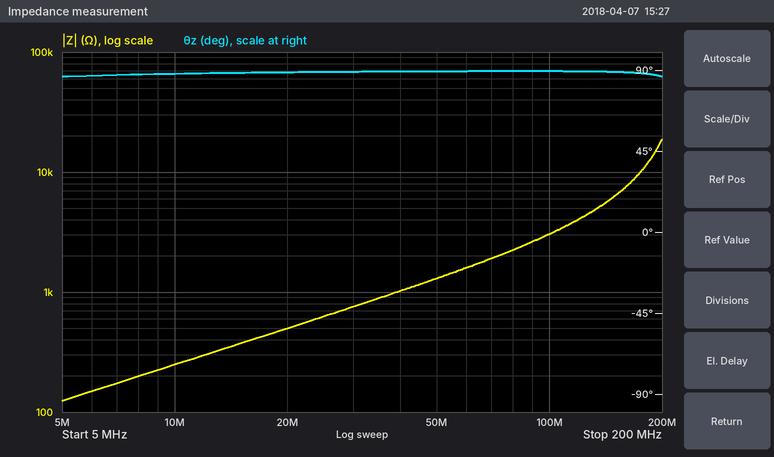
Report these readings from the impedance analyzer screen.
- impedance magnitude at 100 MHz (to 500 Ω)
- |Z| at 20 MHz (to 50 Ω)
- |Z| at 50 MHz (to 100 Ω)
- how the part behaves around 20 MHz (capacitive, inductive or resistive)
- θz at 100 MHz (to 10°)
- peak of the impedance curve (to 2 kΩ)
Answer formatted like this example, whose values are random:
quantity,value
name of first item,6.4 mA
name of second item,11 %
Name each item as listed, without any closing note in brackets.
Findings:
quantity,value
impedance magnitude at 100 MHz,3.0 kΩ
|Z| at 20 MHz,500 Ω
|Z| at 50 MHz,1.3 kΩ
how the part behaves around 20 MHz,inductive
θz at 100 MHz,90°
peak of the impedance curve,18 kΩ
